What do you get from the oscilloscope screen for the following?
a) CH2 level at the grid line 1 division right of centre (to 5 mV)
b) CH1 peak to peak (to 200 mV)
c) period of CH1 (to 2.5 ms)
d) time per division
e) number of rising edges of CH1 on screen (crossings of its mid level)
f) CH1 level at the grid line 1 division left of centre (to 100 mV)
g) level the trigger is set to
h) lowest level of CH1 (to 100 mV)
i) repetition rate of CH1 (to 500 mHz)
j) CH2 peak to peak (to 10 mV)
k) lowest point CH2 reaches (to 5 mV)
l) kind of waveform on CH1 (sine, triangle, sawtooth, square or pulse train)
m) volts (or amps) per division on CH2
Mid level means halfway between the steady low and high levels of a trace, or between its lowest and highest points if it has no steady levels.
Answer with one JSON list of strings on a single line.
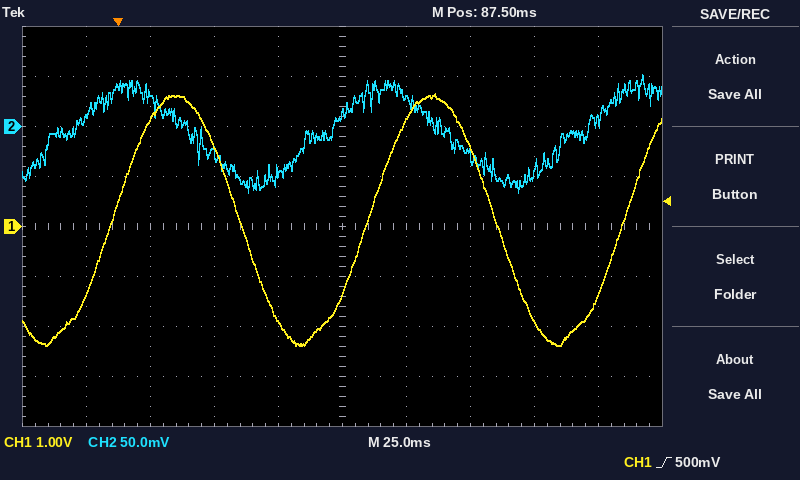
["30 mV", "5.0 V", "100.0 ms", "25 ms", "3", "-1.9 V", "500 mV", "-2.4 V", "10.0 Hz", "120 mV", "-65 mV", "sine", "50 mV"]
